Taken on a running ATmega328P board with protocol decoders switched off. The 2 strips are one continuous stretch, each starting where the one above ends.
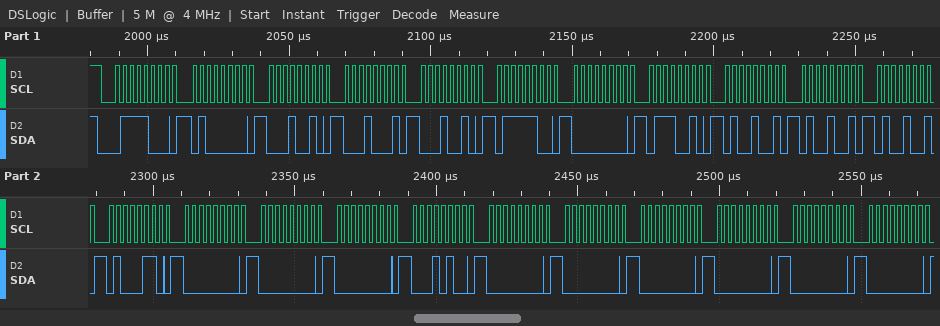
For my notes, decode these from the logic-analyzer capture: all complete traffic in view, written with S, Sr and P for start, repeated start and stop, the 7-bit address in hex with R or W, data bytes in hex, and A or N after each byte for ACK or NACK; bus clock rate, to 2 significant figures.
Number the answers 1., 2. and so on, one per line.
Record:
1. S 3CW A 40 A 12 A 11 A 12 A 7C A 00 A 72 A 49 A 49 A 49 A 46 A 00 A 00 A 00 A 14 A 00 A 00 A 00 A 00 A 00 A 00 A
2. 400 kHz
